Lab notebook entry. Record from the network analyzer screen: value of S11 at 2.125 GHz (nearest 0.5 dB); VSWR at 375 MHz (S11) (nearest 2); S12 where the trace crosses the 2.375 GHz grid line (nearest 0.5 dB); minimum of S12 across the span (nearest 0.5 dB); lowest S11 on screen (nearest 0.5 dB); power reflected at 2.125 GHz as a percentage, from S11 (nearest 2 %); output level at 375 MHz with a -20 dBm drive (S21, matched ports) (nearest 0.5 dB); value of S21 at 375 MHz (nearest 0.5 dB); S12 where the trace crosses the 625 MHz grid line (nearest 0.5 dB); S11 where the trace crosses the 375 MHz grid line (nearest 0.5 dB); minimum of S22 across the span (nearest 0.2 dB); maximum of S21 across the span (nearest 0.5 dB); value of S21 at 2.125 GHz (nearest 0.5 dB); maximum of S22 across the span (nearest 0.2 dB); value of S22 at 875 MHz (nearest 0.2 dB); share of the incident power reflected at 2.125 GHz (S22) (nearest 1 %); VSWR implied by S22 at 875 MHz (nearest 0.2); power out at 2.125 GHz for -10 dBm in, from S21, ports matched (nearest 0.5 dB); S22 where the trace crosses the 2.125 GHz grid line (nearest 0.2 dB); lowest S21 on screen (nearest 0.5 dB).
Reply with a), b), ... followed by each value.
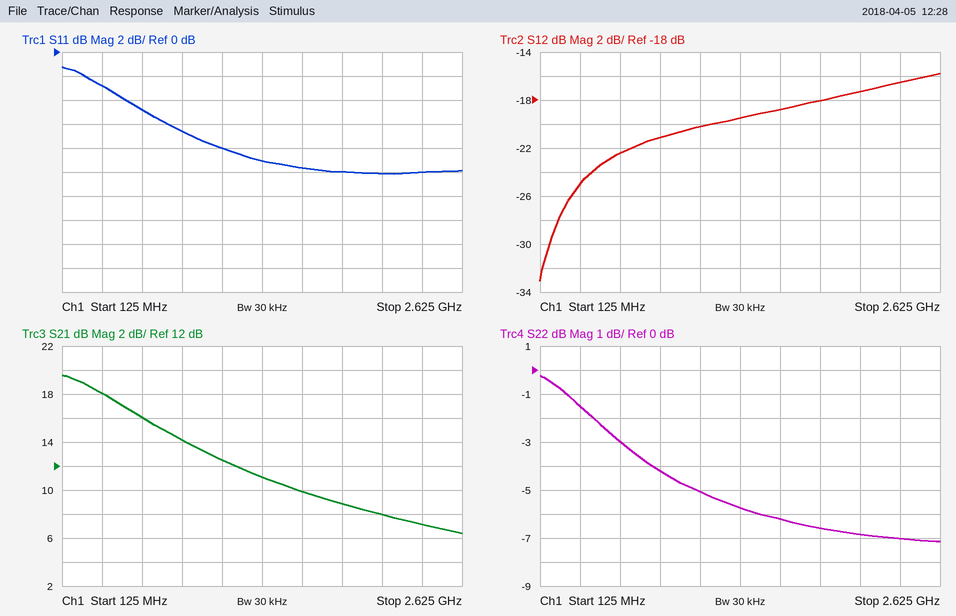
a) -10.0 dB
b) 6
c) -16.5 dB
d) -33.0 dB
e) -10.0 dB
f) 10 %
g) -2.0 dBm
h) 18.0 dB
i) -22.5 dB
j) -3.0 dB
k) -7.2 dB
l) 19.5 dB
m) 8.0 dB
n) -0.2 dB
o) -4.2 dB
p) 21 %
q) 4.2
r) -2.0 dBm
s) -6.8 dB
t) 6.5 dB
